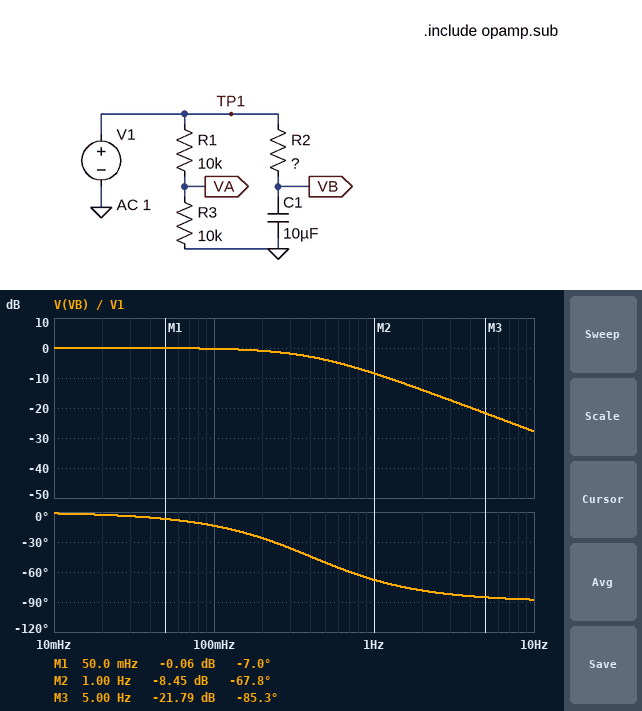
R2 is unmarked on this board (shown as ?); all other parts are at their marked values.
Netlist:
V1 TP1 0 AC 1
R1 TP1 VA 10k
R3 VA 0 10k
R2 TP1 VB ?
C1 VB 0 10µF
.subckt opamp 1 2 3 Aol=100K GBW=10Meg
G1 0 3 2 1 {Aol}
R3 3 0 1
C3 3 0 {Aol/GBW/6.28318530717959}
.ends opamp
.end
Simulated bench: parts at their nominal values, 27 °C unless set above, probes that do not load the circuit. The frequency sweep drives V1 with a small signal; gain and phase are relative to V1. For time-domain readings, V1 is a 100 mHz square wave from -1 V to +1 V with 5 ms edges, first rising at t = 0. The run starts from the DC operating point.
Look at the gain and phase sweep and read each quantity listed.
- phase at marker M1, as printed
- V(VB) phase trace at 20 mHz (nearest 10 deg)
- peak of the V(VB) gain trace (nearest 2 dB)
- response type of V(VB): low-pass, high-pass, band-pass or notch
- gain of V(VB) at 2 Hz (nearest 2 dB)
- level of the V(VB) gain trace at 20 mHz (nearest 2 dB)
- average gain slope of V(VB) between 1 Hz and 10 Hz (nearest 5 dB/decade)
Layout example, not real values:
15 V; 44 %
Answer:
-7.0 deg; 0 deg; 0 dB; low-pass; -14 dB; 0 dB; -20 dB/decade
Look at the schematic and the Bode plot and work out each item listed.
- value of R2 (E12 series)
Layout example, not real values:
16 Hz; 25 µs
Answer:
39 kΩ
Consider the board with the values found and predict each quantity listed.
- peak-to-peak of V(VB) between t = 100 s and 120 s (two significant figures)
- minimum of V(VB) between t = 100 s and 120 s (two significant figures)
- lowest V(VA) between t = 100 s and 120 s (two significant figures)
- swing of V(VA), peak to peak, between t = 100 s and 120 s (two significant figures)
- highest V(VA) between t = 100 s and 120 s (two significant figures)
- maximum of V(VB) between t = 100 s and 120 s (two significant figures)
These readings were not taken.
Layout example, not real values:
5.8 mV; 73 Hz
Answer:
2.0 V; -1.0 V; -500 mV; 1.0 V; 500 mV; 1.0 V
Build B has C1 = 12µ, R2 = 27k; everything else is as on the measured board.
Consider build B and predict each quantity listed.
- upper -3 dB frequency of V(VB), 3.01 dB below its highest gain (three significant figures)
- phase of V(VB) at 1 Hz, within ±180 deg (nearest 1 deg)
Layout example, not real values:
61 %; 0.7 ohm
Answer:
491 mHz; -64 deg
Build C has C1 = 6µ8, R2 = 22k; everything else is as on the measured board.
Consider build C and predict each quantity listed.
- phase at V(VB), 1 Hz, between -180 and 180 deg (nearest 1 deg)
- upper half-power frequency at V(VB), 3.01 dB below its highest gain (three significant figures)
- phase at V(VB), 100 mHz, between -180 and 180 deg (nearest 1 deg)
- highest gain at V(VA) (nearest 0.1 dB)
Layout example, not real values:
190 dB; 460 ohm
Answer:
-43 deg; 1.06 Hz; -5 deg; -6.0 dB
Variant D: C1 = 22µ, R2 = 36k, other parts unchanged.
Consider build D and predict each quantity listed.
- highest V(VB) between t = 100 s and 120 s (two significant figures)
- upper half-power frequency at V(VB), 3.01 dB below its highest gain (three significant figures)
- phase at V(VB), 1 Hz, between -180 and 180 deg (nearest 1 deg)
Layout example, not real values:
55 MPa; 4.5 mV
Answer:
1.0 V; 201 mHz; -79 deg
